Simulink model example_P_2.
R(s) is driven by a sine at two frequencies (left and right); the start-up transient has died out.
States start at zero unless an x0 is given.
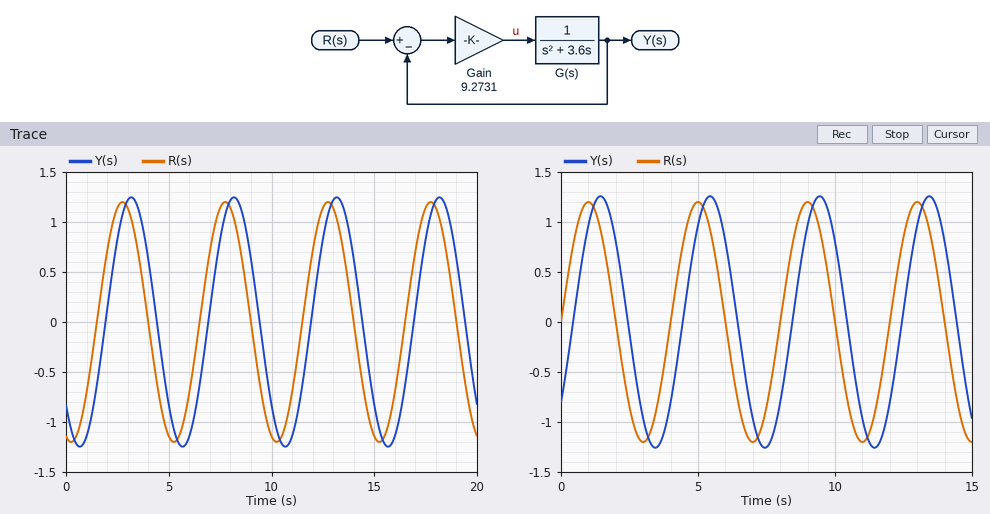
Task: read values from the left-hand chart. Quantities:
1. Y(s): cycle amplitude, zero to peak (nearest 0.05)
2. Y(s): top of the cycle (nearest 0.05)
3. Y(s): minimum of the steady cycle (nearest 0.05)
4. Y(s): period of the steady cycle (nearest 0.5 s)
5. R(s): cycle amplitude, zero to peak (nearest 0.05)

1.25
1.25
-1.25
5.0 s
1.20
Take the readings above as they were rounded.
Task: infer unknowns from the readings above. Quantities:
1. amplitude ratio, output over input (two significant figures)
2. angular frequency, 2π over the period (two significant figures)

1.0
1.3 rad/s
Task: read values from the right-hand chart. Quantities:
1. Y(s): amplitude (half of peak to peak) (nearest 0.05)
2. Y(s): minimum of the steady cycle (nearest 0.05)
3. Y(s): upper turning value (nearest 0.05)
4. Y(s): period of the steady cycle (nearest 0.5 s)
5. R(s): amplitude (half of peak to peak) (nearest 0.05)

1.25
-1.25
1.25
4.0 s
1.20
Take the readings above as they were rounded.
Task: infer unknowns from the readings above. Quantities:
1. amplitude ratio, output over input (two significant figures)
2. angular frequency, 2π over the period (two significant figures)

1.0
1.6 rad/s
